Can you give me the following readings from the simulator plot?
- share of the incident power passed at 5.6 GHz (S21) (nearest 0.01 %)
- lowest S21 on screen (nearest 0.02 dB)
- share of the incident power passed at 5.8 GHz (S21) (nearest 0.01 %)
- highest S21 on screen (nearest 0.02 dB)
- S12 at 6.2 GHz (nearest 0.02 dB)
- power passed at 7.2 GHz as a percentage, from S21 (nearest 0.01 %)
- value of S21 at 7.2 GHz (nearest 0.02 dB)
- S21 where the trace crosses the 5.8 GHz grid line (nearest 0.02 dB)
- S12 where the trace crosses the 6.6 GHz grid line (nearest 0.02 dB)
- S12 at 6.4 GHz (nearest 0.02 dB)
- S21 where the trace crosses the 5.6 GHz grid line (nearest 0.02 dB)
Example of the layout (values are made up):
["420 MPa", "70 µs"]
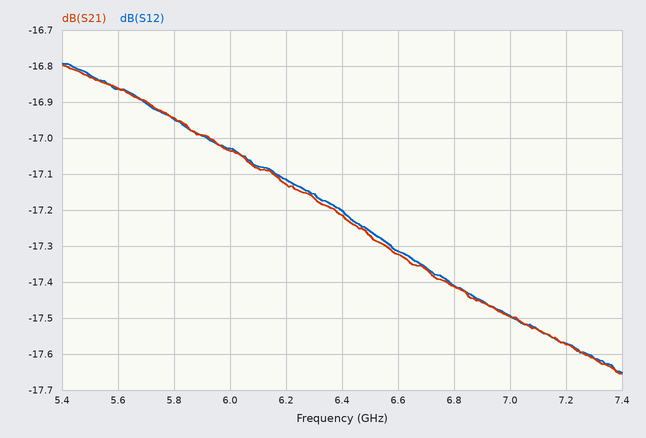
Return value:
["2.06 %", "-17.66 dB", "2.02 %", "-16.80 dB", "-17.12 dB", "1.75 %", "-17.58 dB", "-16.94 dB", "-17.32 dB", "-17.20 dB", "-16.86 dB"]
